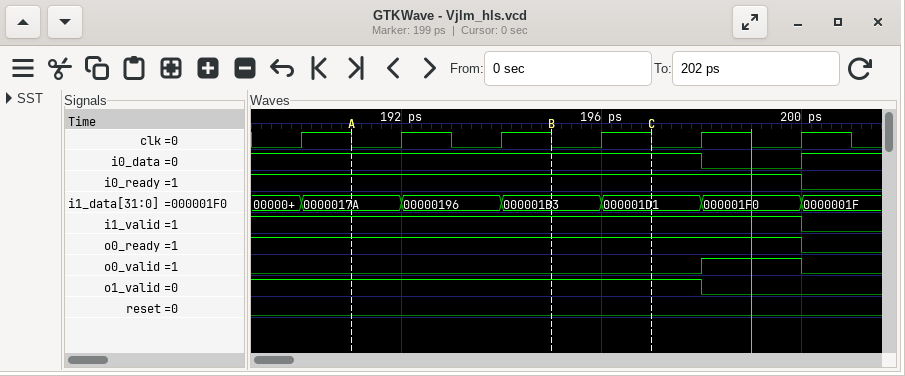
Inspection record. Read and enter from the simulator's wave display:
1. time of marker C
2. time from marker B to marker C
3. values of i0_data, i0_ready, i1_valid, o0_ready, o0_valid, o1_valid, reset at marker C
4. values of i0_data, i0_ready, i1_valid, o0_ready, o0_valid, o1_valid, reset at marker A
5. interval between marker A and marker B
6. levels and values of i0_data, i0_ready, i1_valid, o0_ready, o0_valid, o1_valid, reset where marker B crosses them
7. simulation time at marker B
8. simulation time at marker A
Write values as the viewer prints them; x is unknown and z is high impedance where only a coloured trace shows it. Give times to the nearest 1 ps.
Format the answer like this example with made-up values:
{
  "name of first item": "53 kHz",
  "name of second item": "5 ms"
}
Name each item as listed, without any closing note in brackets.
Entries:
{
  "time of marker C": "197 ps",
  "time from marker B to marker C": "2 ps",
  "values of i0_data, i0_ready, i1_valid, o0_ready, o0_valid, o1_valid, reset at marker C": "i0_data=1, i0_ready=1, i1_valid=1, o0_ready=1, o0_valid=0, o1_valid=1, reset=0",
  "values of i0_data, i0_ready, i1_valid, o0_ready, o0_valid, o1_valid, reset at marker A": "i0_data=1, i0_ready=1, i1_valid=1, o0_ready=1, o0_valid=0, o1_valid=1, reset=0",
  "interval between marker A and marker B": "4 ps",
  "levels and values of i0_data, i0_ready, i1_valid, o0_ready, o0_valid, o1_valid, reset where marker B crosses them": "i0_data=1, i0_ready=1, i1_valid=1, o0_ready=1, o0_valid=0, o1_valid=1, reset=0",
  "simulation time at marker B": "195 ps",
  "simulation time at marker A": "191 ps"
}
